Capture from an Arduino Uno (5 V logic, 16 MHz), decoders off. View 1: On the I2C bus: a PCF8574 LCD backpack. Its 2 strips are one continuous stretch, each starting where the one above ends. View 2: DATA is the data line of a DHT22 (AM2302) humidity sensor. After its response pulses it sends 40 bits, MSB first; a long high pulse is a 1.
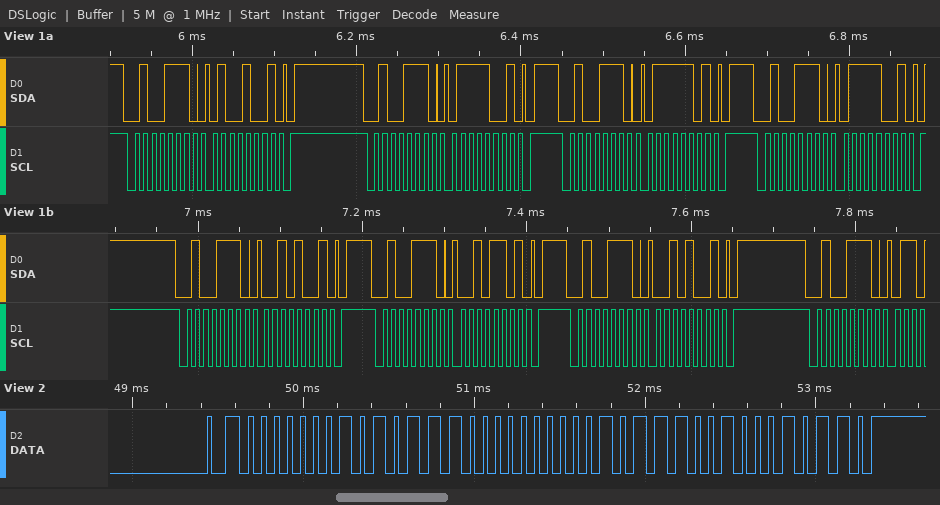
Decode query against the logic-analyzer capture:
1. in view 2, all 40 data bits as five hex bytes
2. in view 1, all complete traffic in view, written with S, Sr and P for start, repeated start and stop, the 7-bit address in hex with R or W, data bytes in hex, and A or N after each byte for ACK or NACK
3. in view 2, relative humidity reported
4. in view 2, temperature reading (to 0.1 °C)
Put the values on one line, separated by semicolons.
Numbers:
01 5C 00 B9 16; S 27W A 49 A P S 27W A 79 A P S 27W A 7D A P S 27W A 79 A P S 27W A 29 A P S 27W A 2D A P S 27W A 29 A P S 27W A; 34.8 %; 18.5 °C
